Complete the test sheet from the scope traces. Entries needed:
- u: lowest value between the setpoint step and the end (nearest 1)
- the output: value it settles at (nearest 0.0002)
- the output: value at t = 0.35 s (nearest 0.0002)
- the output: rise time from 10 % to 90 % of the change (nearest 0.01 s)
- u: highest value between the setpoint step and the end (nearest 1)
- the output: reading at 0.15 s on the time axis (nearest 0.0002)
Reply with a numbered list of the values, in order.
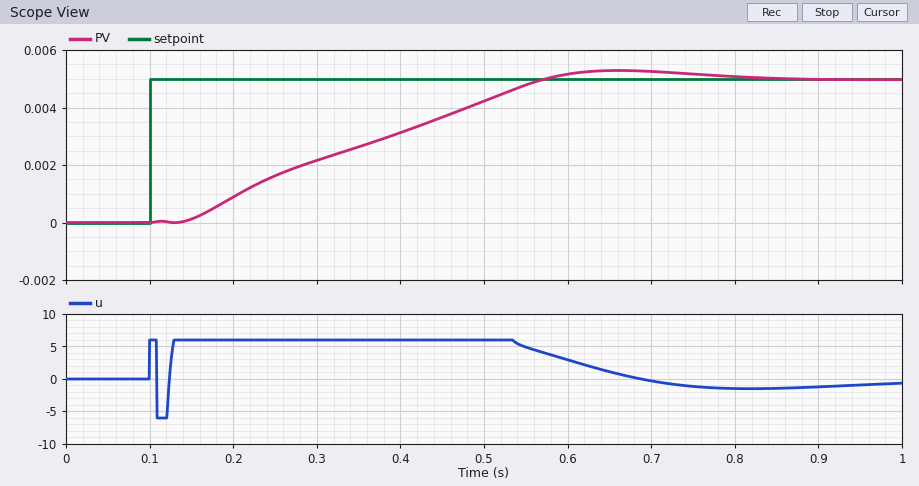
1. -6
2. 0.0050
3. 0.0026
4. 0.35 s
5. 6
6. 0.0002
